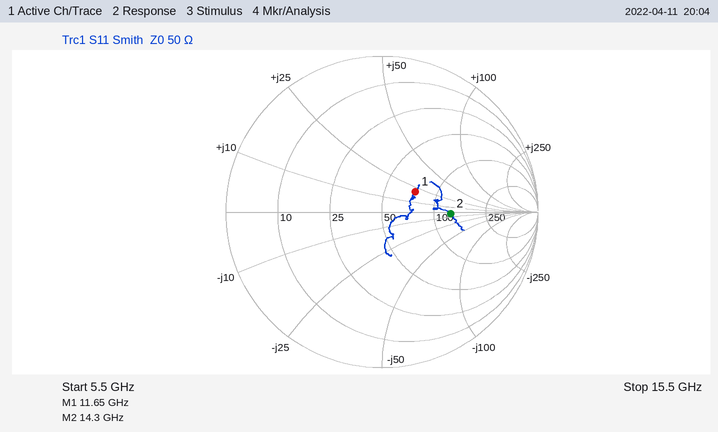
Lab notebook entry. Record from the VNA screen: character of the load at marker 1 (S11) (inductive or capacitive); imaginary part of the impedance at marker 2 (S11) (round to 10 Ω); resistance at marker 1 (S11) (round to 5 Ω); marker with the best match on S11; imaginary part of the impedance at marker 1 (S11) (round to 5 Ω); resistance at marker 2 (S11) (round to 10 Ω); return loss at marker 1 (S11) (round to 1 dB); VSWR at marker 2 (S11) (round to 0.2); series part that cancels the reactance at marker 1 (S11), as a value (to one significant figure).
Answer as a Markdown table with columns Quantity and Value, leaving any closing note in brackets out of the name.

| Quantity | Value |
|---|---|
| character of the load at marker 1 (S11) | inductive |
| imaginary part of the impedance at marker 2 (S11) | 0 Ω |
| resistance at marker 1 (S11) | 75 Ω |
| marker with the best match on S11 | marker 1 |
| imaginary part of the impedance at marker 1 (S11) | +20 Ω |
| resistance at marker 2 (S11) | 130 Ω |
| return loss at marker 1 (S11) | 12 dB |
| VSWR at marker 2 (S11) | 2.6 |
| series part that cancels the reactance at marker 1 (S11), as a value | 700 fF |
